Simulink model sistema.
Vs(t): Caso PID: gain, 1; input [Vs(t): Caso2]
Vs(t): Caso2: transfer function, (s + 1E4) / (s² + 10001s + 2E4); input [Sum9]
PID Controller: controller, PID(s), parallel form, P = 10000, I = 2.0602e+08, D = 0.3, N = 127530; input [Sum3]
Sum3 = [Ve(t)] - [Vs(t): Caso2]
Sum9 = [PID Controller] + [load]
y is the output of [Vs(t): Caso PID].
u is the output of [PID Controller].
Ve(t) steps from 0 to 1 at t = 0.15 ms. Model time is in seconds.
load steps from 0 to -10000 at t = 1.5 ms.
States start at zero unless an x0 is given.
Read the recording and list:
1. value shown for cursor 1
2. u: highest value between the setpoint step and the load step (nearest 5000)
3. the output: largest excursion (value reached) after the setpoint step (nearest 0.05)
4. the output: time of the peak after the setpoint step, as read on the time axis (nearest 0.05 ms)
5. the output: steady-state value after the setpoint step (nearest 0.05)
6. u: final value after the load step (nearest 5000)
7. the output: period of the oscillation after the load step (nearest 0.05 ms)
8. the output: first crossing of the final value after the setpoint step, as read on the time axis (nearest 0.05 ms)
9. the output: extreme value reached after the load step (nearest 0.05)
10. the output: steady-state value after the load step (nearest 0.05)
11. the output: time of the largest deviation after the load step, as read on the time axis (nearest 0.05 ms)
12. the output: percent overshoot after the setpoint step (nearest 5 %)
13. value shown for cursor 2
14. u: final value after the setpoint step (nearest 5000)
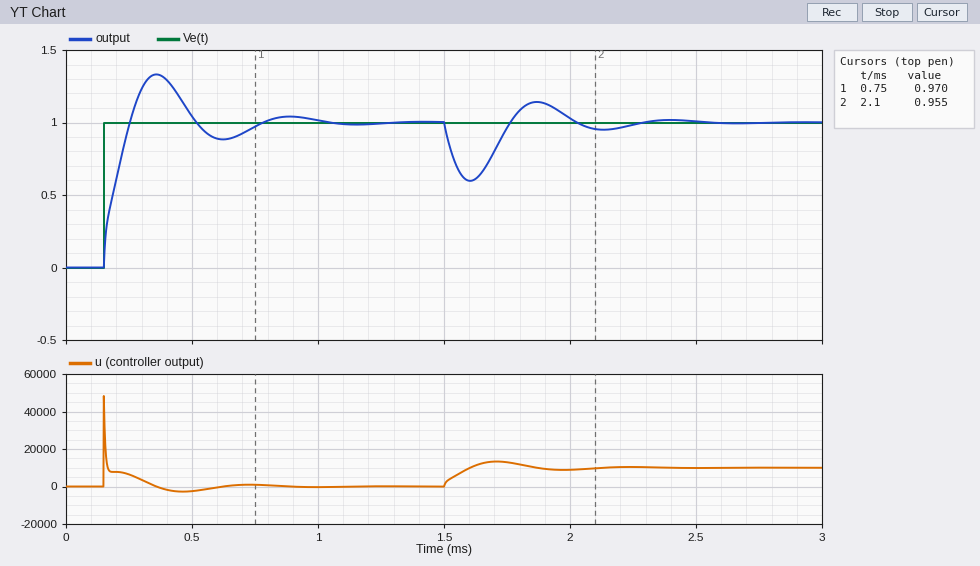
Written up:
0.970
50000
1.35
0.35 ms
1.00
10000
0.55 ms
0.25 ms
0.60
1.00
1.60 ms
35 %
0.955
0
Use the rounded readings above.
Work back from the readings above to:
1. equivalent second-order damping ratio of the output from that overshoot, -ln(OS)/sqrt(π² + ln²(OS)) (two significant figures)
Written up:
0.32
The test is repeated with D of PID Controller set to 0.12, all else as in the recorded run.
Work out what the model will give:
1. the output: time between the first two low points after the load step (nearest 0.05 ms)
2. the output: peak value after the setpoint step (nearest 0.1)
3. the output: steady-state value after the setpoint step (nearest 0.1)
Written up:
0.50 ms
1.4
1.0
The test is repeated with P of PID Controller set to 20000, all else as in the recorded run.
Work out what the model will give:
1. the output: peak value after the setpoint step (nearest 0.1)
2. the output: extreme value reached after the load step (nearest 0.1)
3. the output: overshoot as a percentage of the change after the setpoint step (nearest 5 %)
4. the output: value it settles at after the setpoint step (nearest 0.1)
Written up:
1.2
0.7
20 %
1.0
